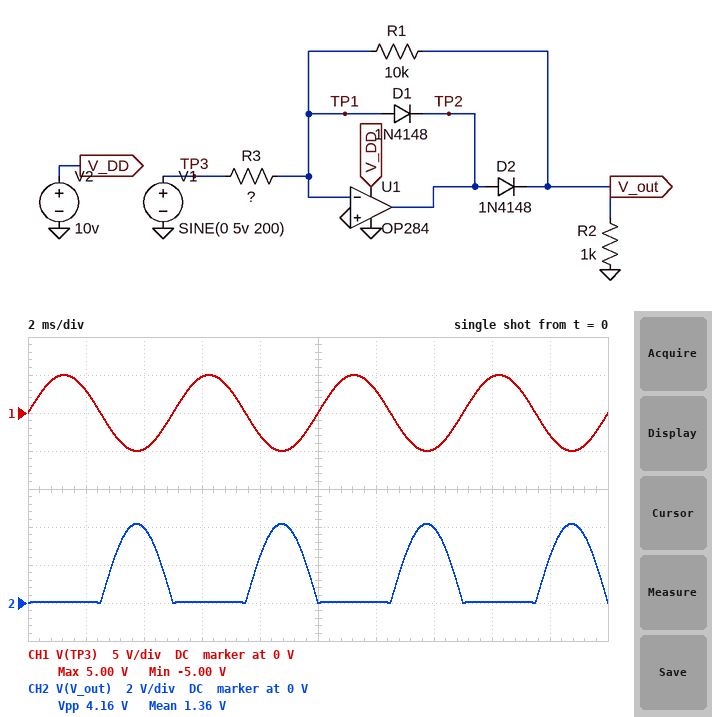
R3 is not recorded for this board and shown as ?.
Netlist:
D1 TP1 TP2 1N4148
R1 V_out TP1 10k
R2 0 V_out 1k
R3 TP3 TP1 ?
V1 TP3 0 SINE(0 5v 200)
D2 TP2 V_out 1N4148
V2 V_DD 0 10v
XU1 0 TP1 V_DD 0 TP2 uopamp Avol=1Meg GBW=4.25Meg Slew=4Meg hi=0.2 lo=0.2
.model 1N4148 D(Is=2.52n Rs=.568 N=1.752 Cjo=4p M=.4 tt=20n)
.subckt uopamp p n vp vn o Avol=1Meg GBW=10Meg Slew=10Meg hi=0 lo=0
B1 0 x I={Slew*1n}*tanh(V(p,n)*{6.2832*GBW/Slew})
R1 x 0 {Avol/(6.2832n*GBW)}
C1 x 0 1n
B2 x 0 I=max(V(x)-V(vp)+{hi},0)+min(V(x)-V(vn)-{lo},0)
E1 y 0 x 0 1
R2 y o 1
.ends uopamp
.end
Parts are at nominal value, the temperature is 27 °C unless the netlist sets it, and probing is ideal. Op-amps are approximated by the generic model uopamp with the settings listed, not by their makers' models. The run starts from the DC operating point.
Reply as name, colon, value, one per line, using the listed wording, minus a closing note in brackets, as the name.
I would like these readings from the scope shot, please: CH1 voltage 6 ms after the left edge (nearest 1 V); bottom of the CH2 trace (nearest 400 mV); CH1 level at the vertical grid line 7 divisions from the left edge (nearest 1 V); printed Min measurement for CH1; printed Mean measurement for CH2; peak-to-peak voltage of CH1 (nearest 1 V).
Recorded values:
CH1 voltage 6 ms after the left edge: 5 V
bottom of the CH2 trace: 0 V
CH1 level at the vertical grid line 7 divisions from the left edge: -5 V
printed Min measurement for CH1: -5.00 V
printed Mean measurement for CH2: 1.36 V
peak-to-peak voltage of CH1: 10 V
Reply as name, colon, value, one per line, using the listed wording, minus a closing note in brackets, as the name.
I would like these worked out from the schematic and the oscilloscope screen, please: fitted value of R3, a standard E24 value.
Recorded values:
fitted value of R3, a standard E24 value: 12 kΩ
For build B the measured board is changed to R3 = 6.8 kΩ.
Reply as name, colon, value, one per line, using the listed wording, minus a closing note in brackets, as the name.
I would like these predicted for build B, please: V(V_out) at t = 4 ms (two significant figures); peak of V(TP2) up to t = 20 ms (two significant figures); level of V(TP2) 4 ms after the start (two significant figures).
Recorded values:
V(V_out) at t = 4 ms: 7.0 V
peak of V(TP2) up to t = 20 ms: 8.0 V
level of V(TP2) 4 ms after the start: 7.7 V
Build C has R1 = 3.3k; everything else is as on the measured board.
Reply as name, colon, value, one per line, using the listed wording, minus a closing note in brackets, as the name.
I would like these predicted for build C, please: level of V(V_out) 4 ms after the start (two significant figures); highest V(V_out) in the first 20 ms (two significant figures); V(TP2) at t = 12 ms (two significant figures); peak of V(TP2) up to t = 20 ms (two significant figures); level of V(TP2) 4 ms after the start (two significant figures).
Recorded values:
level of V(V_out) 4 ms after the start: 1.3 V
highest V(V_out) in the first 20 ms: 1.4 V
V(TP2) at t = 12 ms: 200 mV
peak of V(TP2) up to t = 20 ms: 2.0 V
level of V(TP2) 4 ms after the start: 1.9 V
